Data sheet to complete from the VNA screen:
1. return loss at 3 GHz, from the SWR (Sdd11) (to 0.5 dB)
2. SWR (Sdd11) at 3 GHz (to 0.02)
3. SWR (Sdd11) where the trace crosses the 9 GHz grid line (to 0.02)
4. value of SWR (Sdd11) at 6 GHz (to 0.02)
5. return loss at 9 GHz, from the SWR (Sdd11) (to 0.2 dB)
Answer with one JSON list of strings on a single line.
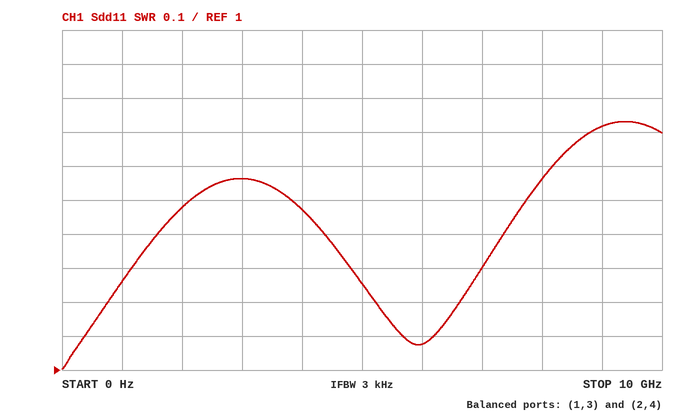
["13.0 dB", "1.56", "1.72", "1.08", "11.6 dB"]
